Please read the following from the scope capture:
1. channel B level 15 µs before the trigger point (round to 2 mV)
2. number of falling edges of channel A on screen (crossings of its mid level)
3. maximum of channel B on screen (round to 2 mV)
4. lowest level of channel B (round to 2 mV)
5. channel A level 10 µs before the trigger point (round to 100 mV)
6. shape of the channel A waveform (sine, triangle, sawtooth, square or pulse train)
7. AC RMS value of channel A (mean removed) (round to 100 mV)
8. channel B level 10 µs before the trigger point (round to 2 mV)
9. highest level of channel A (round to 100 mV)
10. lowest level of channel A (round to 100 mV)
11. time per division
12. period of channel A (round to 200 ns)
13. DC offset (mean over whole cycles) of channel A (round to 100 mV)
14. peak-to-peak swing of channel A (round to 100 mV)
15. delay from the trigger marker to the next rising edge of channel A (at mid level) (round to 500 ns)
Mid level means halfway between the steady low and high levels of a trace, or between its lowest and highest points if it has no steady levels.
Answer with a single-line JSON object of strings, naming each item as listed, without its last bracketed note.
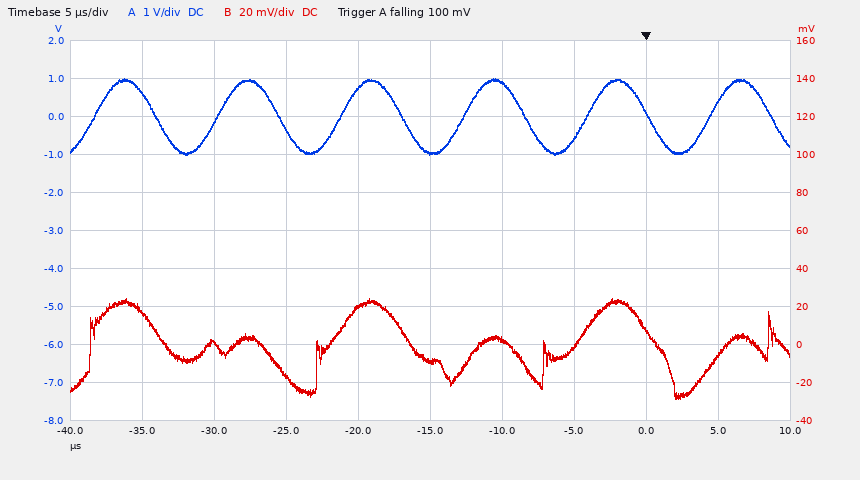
{"channel B level 15 µs before the trigger point": "-8 mV", "number of falling edges of channel A on screen": "6", "maximum of channel B on screen": "24 mV", "lowest level of channel B": "-28 mV", "channel A level 10 µs before the trigger point": "900 mV", "shape of the channel A waveform": "sine", "AC RMS value of channel A (mean removed)": "700 mV", "channel B level 10 µs before the trigger point": "2 mV", "highest level of channel A": "1.0 V", "lowest level of channel A": "-1.0 V", "time per division": "5 µs", "period of channel A": "8.6 µs", "DC offset (mean over whole cycles) of channel A": "0.0 V", "peak-to-peak swing of channel A": "2.0 V", "delay from the trigger marker to the next rising edge of channel A (at mid level)": "4.5 µs"}
